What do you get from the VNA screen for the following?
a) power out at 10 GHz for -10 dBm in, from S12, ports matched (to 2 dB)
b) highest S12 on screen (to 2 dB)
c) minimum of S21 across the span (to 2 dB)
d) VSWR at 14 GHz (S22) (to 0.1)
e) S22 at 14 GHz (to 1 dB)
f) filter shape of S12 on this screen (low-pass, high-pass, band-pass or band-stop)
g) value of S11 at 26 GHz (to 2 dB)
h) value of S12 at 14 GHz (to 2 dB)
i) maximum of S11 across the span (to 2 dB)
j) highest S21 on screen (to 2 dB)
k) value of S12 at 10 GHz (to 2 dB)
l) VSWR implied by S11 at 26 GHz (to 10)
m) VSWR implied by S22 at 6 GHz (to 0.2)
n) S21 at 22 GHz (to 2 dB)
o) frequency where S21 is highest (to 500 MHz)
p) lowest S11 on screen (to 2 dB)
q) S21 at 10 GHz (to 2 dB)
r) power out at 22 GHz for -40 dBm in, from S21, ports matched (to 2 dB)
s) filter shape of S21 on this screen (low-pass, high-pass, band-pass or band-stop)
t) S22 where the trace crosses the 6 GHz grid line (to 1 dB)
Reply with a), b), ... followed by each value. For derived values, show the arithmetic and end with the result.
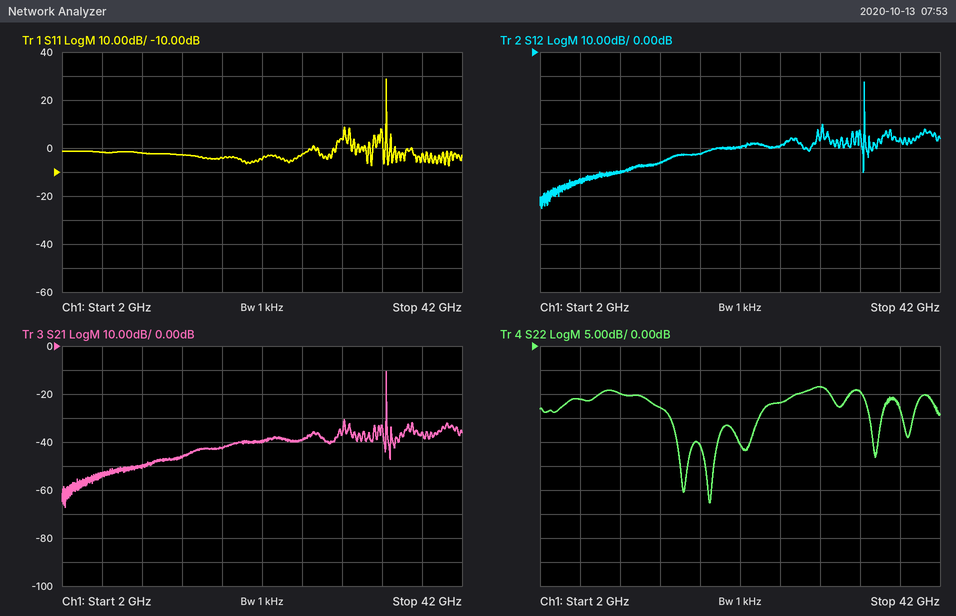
a) -10 dBm + (-50 dB) = -60 dBm
b) -12 dB
c) -68 dB
d) |Γ| = 10^(-13/20) = 0.2239; VSWR = (1 + 0.2239)/(1 − 0.2239) ≈ 1.6
e) -13 dB
f) band-pass
g) -2 dB
h) -46 dB
i) 28 dB
j) -10 dB
k) -50 dB
l) |Γ| = 10^(-2/20) = 0.7943; VSWR = (1 + 0.7943)/(1 − 0.7943) ≈ 8.72, so 10 to the nearest 10
m) |Γ| = 10^(-11/20) = 0.2818; VSWR = (1 + 0.2818)/(1 − 0.2818) ≈ 1.8
n) -40 dB
o) 34.5 GHz
p) -8 dB
q) -50 dB
r) -40 dBm + (-40 dB) = -80 dBm
s) band-pass
t) -11 dB
